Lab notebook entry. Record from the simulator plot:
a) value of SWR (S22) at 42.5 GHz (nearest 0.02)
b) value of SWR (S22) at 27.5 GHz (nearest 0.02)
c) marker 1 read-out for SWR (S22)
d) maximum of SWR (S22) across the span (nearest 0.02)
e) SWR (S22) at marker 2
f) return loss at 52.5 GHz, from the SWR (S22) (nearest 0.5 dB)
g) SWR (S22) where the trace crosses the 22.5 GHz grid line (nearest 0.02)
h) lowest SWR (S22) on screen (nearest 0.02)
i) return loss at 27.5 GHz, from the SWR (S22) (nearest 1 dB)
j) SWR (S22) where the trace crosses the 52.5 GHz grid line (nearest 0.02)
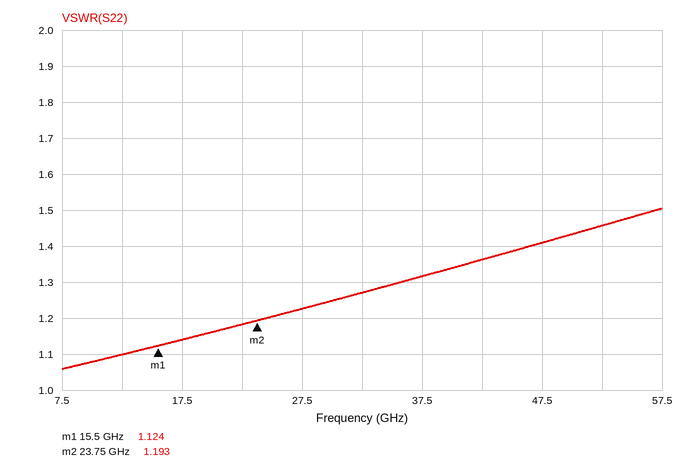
1.36
1.22
1.124
1.50
1.193
14.5 dB
1.18
1.06
20 dB
1.46
